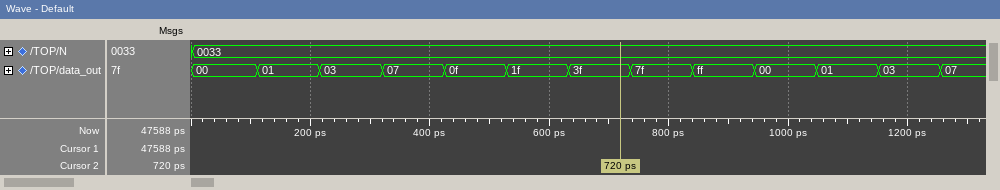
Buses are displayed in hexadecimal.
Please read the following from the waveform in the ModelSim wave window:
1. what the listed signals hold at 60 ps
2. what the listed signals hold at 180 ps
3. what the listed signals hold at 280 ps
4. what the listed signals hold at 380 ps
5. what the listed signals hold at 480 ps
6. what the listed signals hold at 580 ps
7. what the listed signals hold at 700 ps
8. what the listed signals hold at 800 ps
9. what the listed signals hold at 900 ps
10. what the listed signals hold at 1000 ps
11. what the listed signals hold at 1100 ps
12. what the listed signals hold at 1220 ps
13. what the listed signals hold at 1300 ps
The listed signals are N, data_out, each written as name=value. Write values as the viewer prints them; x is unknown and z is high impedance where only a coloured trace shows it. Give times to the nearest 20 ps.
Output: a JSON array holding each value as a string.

["N=0033, data_out=00", "N=0033, data_out=01", "N=0033, data_out=03", "N=0033, data_out=07", "N=0033, data_out=0f", "N=0033, data_out=1f", "N=0033, data_out=3f", "N=0033, data_out=7f", "N=0033, data_out=ff", "N=0033, data_out=00", "N=0033, data_out=01", "N=0033, data_out=03", "N=0033, data_out=07"]
